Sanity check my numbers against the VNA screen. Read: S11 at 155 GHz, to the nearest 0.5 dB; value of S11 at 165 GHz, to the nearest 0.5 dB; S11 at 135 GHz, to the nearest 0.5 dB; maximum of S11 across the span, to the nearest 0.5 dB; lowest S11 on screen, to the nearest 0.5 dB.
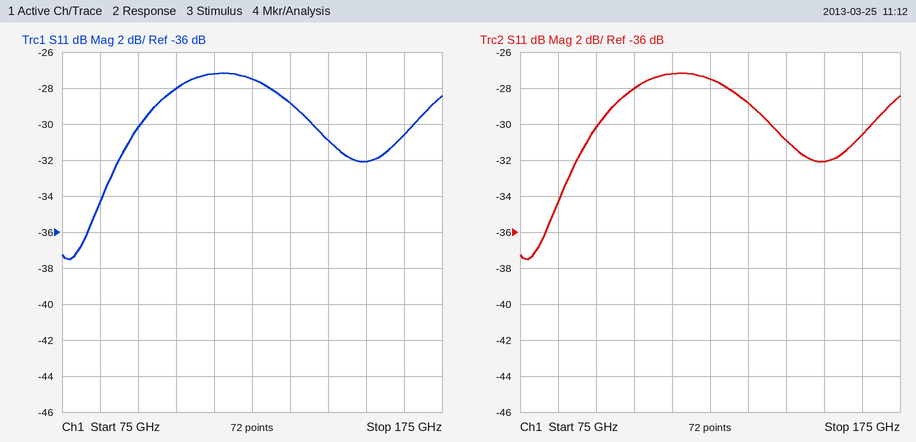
-32.0 dB
-30.5 dB
-29.0 dB
-27.0 dB
-37.5 dB
